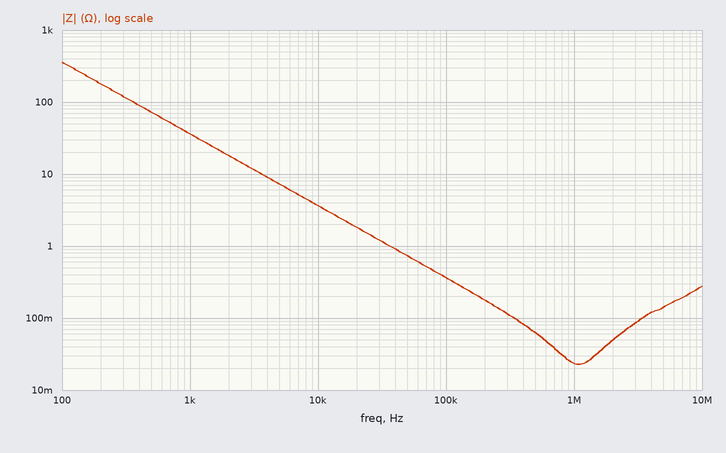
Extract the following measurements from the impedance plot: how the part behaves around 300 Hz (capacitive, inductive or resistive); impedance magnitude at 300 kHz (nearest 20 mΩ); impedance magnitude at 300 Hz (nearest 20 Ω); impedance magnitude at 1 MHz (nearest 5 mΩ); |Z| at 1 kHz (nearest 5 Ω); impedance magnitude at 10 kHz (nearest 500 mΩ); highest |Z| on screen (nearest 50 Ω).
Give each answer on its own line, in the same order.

capacitive
120 mΩ
120 Ω
25 mΩ
35 Ω
3.5 Ω
350 Ω
